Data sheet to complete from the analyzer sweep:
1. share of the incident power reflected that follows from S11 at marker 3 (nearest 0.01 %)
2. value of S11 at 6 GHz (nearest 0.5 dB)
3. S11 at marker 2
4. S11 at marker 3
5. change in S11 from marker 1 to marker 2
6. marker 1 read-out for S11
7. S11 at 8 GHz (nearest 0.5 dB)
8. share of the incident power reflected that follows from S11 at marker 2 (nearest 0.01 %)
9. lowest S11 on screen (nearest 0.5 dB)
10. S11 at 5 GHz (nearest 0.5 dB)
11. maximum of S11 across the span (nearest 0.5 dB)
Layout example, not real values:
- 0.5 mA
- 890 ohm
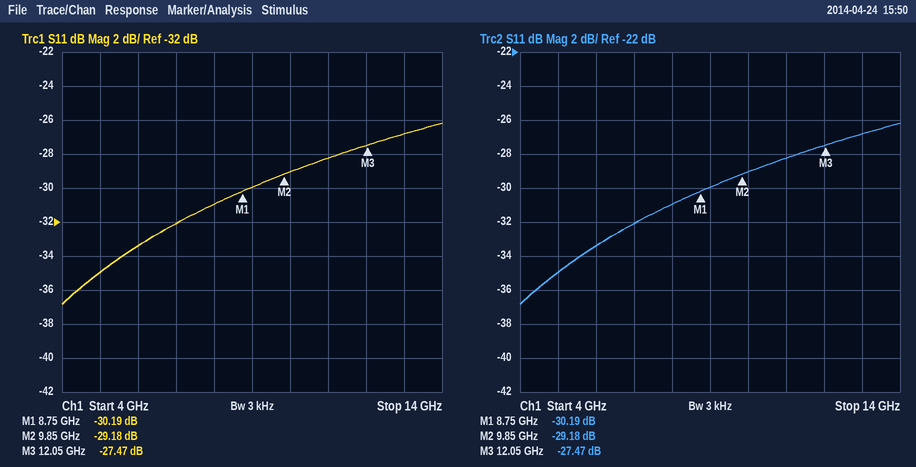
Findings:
- 0.18 %
- -33.5 dB
- -29.18 dB
- -27.47 dB
- 1.01 dB
- -30.19 dB
- -31.0 dB
- 0.12 %
- -37.0 dB
- -35.0 dB
- -26.0 dB
